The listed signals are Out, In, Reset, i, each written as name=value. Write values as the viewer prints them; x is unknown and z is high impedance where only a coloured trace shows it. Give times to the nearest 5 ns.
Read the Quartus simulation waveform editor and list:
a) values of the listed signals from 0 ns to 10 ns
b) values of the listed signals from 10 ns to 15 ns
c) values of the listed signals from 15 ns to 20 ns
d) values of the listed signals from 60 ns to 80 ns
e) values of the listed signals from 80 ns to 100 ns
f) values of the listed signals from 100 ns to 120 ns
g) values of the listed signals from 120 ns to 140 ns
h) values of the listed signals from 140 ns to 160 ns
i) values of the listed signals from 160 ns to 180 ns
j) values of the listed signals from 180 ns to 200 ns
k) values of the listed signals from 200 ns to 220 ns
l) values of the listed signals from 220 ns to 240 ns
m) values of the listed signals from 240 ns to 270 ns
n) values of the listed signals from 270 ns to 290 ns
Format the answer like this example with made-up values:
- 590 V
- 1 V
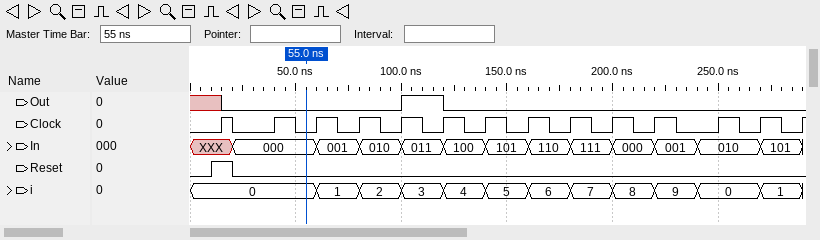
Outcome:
- Out=x, In=XXX, Reset=0, i=0
- Out=x, In=XXX, Reset=1, i=0
- Out=0, In=XXX, Reset=1, i=0
- Out=0, In=001, Reset=0, i=1
- Out=0, In=010, Reset=0, i=2
- Out=1, In=011, Reset=0, i=3
- Out=0, In=100, Reset=0, i=4
- Out=0, In=101, Reset=0, i=5
- Out=0, In=110, Reset=0, i=6
- Out=0, In=111, Reset=0, i=7
- Out=0, In=000, Reset=0, i=8
- Out=0, In=001, Reset=0, i=9
- Out=0, In=010, Reset=0, i=0
- Out=0, In=101, Reset=0, i=1
